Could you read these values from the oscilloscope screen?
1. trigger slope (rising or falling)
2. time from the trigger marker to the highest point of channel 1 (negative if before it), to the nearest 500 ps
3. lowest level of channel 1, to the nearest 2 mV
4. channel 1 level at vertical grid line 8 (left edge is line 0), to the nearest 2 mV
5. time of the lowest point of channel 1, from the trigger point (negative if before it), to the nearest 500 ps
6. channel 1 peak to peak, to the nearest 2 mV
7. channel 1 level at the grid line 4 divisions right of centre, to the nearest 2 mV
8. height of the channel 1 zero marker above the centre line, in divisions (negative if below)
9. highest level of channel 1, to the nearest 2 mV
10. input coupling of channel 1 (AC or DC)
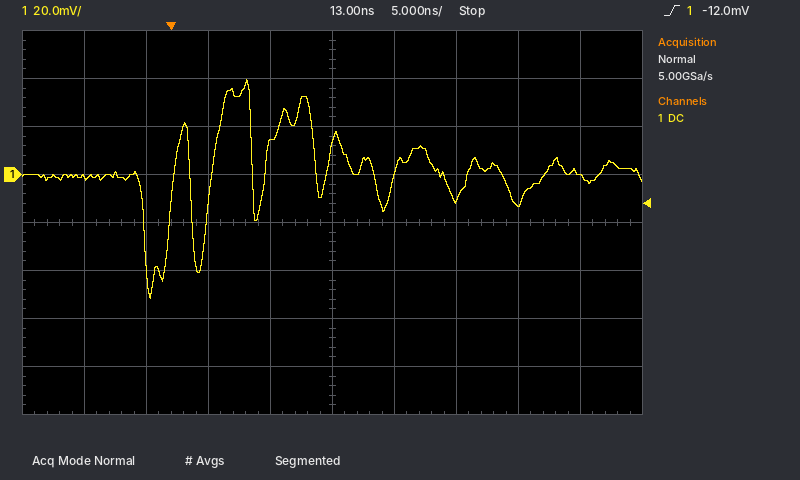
rising
+6.0 ns
-52 mV
-12 mV
-1.5 ns
92 mV
0 mV
+1.0 div
40 mV
DC
